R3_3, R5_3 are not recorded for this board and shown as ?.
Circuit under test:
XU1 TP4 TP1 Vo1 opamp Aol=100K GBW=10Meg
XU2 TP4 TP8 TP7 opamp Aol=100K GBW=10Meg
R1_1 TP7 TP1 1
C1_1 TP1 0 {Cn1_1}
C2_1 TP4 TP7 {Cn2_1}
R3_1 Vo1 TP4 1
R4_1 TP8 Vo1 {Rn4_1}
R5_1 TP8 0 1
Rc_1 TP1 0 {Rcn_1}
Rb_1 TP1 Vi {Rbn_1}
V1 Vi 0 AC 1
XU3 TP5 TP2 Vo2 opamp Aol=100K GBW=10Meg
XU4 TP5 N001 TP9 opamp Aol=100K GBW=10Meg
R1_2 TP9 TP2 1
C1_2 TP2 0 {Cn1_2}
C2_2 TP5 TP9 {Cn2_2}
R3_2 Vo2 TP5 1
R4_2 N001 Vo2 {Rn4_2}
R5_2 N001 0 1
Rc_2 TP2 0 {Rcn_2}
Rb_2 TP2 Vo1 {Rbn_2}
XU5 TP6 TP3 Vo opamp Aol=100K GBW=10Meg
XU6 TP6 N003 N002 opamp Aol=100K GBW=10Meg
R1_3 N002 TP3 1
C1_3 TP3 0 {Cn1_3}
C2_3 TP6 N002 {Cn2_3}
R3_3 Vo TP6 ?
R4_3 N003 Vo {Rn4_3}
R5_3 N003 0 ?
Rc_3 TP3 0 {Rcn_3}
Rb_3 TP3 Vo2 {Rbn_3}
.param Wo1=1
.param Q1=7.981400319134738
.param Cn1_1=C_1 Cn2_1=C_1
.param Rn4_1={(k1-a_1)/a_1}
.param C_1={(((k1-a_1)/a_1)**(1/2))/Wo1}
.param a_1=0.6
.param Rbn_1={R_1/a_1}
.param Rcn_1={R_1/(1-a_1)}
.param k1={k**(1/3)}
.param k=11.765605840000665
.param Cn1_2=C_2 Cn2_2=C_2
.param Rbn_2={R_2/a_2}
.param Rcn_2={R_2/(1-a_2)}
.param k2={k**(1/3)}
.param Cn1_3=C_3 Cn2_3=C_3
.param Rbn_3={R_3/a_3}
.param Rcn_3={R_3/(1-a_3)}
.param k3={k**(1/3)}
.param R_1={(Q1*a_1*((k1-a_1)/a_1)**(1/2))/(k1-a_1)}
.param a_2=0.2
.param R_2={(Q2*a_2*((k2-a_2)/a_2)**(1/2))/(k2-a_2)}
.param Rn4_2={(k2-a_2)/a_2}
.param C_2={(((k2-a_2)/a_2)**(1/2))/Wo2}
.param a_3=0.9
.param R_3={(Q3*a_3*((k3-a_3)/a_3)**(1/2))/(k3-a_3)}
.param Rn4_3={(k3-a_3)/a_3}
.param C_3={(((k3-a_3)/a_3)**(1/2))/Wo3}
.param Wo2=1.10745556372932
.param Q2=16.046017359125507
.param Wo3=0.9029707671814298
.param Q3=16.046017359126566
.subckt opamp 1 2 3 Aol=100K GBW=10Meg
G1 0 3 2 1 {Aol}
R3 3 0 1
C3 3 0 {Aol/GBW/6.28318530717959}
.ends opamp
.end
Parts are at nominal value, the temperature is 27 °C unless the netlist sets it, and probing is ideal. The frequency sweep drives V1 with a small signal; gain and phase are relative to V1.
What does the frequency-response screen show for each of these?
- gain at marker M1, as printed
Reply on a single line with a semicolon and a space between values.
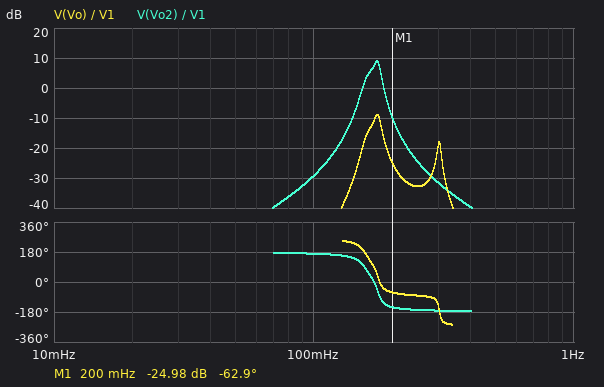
-24.98 dB
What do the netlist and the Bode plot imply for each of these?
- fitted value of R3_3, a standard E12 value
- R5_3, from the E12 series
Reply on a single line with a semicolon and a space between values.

0.68 Ω; 0.33 Ω
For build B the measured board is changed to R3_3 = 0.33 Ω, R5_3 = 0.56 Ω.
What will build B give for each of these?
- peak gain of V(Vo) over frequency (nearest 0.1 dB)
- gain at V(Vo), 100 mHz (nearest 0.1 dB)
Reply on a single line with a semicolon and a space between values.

-14.9 dB; -59.8 dB
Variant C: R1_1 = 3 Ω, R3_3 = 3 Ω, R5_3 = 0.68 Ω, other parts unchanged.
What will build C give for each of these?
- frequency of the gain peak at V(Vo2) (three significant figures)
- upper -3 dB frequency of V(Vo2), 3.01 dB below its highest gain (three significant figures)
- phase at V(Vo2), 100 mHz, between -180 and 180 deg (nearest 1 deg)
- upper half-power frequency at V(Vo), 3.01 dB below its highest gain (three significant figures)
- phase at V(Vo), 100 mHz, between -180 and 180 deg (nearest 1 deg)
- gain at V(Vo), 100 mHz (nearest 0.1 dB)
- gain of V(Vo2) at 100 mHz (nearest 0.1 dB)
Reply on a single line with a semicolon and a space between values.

176 mHz; 181 mHz; 49 deg; 104 mHz; 57 deg; -4.2 dB; -13.5 dB
